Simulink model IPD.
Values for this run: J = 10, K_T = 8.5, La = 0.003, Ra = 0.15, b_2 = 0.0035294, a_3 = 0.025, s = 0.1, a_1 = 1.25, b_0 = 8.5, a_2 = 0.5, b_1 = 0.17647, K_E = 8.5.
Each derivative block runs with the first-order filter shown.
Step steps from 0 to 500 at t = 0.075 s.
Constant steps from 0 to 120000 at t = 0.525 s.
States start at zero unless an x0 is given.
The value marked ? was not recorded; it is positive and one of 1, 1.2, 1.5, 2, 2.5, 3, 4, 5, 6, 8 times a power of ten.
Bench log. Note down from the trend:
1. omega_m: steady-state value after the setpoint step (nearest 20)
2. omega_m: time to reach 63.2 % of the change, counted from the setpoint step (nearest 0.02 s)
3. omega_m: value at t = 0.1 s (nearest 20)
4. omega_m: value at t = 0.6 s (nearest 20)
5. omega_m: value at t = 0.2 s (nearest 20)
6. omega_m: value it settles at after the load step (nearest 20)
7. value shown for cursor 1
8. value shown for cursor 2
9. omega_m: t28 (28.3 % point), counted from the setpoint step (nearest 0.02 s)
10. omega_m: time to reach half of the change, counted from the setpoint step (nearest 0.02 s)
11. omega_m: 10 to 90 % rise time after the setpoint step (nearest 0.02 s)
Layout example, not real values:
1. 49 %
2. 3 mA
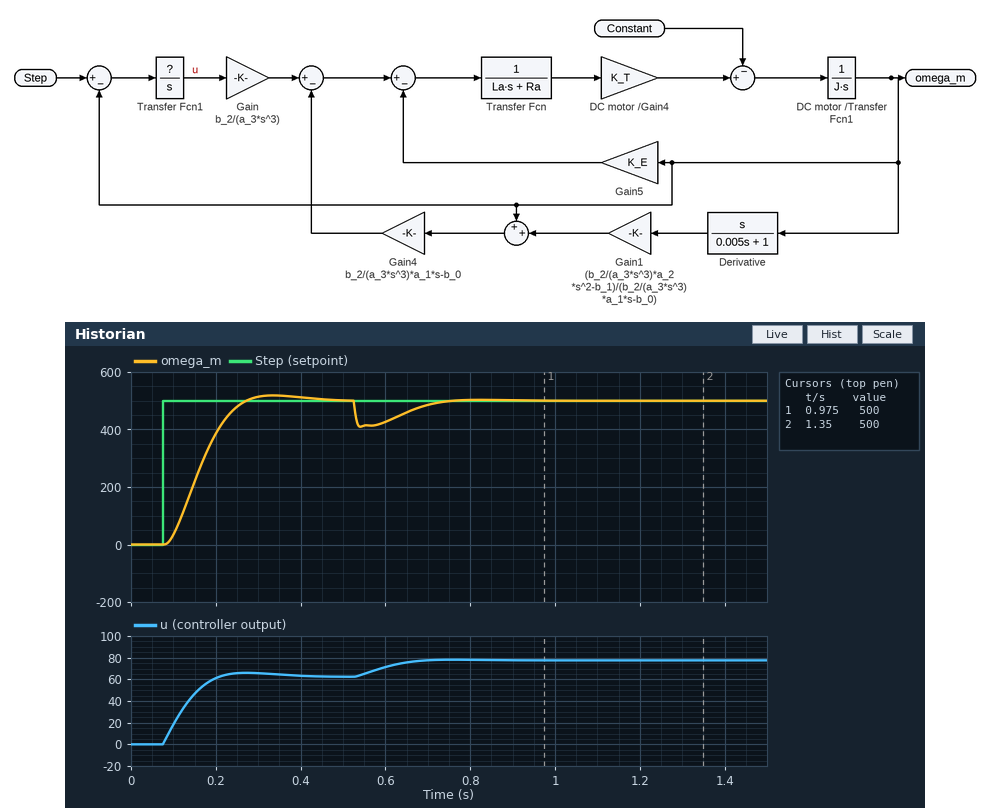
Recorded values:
1. 500
2. 0.10 s
3. 40
4. 420
5. 380
6. 500
7. 500
8. 500
9. 0.06 s
10. 0.08 s
11. 0.12 s
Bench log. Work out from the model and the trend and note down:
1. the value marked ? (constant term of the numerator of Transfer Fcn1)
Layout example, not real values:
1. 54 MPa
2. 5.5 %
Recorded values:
1. 1.5
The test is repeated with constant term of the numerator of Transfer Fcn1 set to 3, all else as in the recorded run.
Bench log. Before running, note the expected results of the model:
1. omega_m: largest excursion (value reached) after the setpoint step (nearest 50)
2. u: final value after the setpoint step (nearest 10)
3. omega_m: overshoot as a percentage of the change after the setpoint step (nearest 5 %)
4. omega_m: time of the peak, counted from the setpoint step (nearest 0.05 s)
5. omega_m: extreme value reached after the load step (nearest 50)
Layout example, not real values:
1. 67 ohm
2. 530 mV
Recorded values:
1. 600
2. 60
3. 15 %
4. 0.15 s
5. 400
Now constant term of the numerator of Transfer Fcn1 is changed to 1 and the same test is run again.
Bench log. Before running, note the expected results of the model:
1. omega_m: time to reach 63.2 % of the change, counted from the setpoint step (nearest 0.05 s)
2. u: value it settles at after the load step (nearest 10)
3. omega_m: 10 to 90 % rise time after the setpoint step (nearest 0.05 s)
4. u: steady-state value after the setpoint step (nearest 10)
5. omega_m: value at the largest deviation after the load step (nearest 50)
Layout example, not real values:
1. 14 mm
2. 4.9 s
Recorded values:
1. 0.15 s
2. 80
3. 0.20 s
4. 60
5. 400
